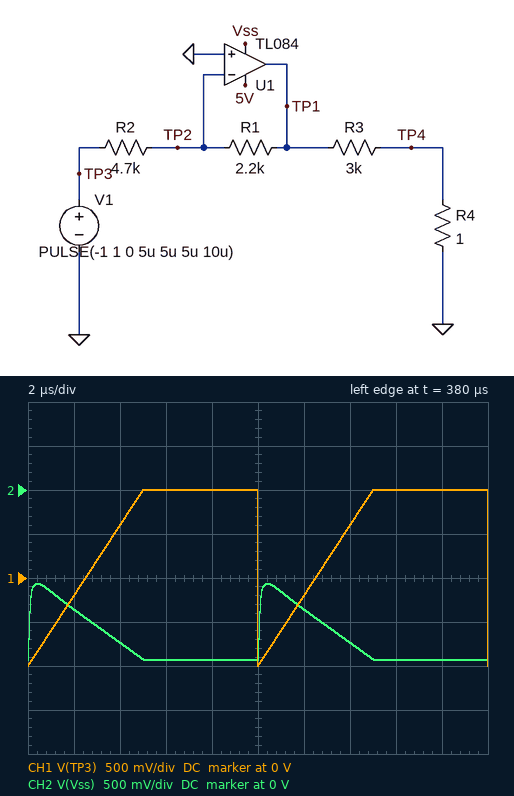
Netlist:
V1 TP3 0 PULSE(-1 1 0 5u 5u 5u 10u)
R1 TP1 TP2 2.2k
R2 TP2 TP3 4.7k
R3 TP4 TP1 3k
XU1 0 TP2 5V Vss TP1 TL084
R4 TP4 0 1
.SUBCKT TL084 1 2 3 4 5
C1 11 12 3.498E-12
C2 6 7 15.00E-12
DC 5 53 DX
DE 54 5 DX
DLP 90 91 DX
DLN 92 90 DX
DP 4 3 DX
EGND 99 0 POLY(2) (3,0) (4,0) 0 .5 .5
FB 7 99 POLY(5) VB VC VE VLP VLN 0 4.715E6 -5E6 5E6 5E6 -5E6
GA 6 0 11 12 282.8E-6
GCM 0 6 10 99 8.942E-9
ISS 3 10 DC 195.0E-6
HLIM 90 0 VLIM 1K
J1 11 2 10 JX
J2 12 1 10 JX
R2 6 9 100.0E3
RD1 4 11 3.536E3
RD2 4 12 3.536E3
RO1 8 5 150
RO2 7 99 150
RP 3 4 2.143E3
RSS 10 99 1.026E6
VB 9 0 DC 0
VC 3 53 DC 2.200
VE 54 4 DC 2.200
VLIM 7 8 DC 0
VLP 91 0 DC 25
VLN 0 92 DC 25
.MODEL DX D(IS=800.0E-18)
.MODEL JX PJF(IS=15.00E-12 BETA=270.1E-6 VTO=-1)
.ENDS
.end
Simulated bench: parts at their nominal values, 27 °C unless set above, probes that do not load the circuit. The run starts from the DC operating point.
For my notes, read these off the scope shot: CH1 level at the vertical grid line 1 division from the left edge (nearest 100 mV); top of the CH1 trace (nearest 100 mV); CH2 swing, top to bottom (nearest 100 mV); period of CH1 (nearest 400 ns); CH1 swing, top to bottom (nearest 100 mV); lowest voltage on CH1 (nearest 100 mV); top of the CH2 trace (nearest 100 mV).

-200 mV
1.0 V
900 mV
10.0 µs
2.0 V
-1.0 V
-1.1 V
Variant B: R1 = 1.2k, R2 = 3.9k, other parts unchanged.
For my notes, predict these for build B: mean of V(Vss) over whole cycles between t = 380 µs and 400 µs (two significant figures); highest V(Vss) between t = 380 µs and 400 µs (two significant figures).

-1.6 V
-1.2 V
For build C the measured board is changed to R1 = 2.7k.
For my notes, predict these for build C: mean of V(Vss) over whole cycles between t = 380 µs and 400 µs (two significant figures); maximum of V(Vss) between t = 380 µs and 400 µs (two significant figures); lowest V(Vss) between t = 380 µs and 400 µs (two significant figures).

-1.8 V
-990 mV
-2.0 V
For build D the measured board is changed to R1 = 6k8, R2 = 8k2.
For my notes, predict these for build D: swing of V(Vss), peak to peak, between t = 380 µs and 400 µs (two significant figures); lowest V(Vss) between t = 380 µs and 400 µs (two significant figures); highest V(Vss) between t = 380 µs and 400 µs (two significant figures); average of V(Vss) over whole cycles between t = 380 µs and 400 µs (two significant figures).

1.5 V
-2.3 V
-840 mV
-1.9 V
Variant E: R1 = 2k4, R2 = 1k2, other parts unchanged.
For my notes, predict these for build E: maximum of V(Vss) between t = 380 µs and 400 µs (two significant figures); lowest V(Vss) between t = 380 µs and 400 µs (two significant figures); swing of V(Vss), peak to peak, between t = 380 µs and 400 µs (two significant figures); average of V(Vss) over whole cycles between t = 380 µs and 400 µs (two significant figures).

-430 mV
-3.5 V
3.1 V
-2.5 V
